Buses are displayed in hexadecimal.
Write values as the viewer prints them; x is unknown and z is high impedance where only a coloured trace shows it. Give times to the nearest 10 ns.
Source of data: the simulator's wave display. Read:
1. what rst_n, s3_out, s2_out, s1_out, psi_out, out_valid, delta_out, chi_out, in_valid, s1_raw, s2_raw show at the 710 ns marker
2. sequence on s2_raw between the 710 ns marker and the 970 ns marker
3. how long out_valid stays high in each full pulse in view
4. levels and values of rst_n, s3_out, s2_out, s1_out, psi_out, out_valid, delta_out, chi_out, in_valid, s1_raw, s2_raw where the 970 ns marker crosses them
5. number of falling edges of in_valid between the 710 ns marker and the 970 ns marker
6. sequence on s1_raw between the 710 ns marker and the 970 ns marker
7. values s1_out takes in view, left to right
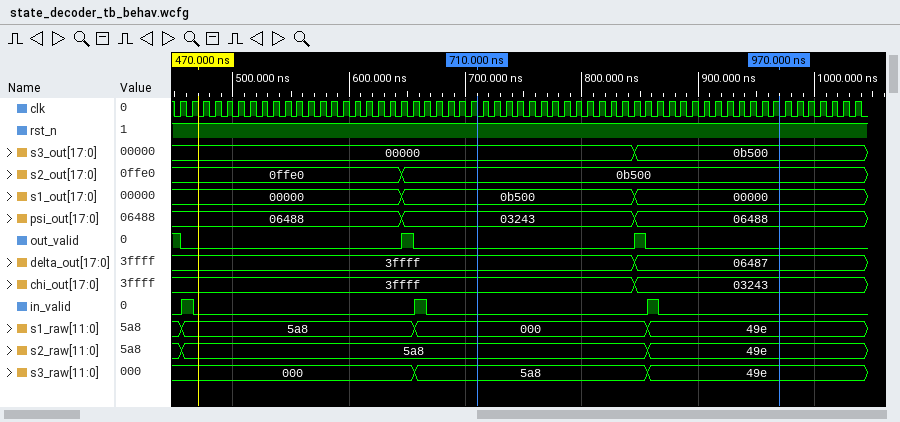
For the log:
rst_n=1, s3_out=00000, s2_out=0b500, s1_out=0b500, psi_out=03243, out_valid=0, delta_out=3ffff, chi_out=3ffff, in_valid=0, s1_raw=000, s2_raw=5a8
5a8, 49e
10 ns, 10 ns
rst_n=1, s3_out=0b500, s2_out=0b500, s1_out=00000, psi_out=06488, out_valid=0, delta_out=06487, chi_out=03243, in_valid=0, s1_raw=49e, s2_raw=49e
1
000, 49e
00000, 0b500, 00000
